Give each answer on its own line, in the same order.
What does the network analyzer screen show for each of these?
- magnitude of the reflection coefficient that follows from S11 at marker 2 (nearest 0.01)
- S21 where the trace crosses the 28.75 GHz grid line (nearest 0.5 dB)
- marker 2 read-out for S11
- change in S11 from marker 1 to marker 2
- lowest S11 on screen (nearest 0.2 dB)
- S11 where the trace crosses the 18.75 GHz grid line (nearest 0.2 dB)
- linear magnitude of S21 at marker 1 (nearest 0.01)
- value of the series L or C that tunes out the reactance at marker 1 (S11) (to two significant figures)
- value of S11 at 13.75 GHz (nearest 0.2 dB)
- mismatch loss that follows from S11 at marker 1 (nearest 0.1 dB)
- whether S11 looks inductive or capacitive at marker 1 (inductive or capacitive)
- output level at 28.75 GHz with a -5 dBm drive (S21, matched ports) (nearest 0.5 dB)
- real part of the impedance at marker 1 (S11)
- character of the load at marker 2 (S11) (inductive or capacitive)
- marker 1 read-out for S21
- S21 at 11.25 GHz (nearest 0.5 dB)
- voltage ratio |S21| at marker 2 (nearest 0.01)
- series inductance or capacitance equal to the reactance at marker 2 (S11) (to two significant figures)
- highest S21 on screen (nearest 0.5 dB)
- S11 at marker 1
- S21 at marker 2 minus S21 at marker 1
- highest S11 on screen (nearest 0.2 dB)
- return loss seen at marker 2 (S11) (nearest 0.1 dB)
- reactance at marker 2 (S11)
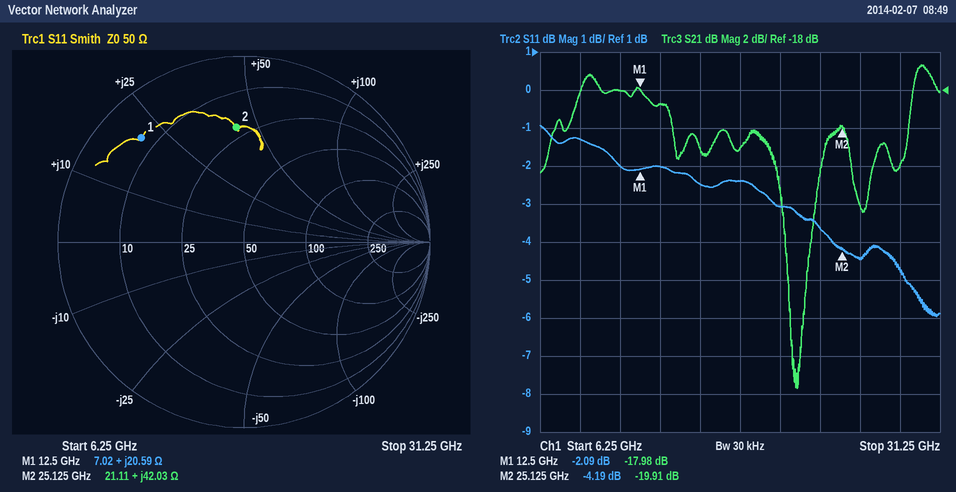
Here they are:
0.62
-22.0 dB
-4.19 dB
-2.10 dB
-6.0 dB
-2.4 dB
0.13
620 fF
-2.0 dB
4.2 dB
inductive
-27.0 dBm
7.02 Ω
inductive
-17.98 dB
-18.0 dB
0.10
270 pH
-16.5 dB
-2.09 dB
-1.93 dB
-1.0 dB
4.2 dB
+42.03 Ω
